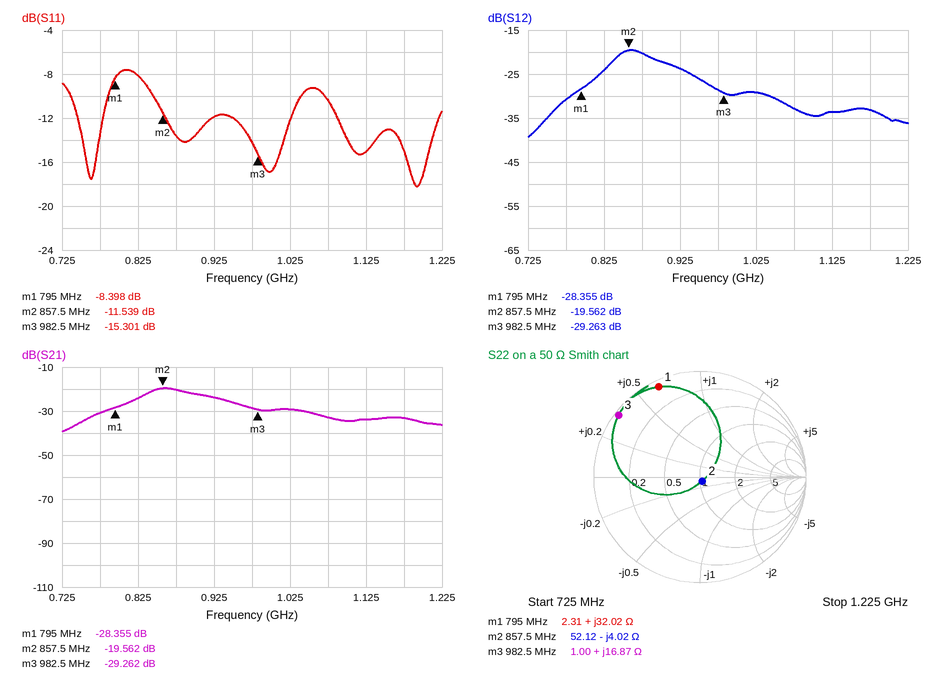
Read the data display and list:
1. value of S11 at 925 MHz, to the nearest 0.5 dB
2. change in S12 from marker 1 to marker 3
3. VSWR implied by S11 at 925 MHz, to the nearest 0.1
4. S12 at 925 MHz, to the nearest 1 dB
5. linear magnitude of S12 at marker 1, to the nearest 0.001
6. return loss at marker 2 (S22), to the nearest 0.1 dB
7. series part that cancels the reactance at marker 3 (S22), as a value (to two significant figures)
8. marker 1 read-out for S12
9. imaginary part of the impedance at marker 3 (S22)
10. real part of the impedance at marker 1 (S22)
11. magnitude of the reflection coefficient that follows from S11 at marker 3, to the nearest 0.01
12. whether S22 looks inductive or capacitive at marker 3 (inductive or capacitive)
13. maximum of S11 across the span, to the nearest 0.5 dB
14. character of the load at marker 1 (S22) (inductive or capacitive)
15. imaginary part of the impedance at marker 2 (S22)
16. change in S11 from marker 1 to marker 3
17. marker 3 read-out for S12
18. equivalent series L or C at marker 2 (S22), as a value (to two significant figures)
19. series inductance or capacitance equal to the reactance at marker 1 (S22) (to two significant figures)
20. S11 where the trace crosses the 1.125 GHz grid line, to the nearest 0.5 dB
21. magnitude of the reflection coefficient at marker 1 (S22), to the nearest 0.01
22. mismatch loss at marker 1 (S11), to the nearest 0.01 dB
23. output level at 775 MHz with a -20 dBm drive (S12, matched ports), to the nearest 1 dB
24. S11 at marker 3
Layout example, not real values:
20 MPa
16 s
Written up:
-12.0 dB
-0.908 dB
1.7
-24 dB
0.038
27.0 dB
9.6 pF
-28.355 dB
+16.87 Ω
2.31 Ω
0.17
inductive
-7.5 dB
inductive
-4.02 Ω
-6.903 dB
-29.263 dB
46 pF
6.4 nH
-15.0 dB
0.94
0.68 dB
-51 dBm
-15.301 dB
